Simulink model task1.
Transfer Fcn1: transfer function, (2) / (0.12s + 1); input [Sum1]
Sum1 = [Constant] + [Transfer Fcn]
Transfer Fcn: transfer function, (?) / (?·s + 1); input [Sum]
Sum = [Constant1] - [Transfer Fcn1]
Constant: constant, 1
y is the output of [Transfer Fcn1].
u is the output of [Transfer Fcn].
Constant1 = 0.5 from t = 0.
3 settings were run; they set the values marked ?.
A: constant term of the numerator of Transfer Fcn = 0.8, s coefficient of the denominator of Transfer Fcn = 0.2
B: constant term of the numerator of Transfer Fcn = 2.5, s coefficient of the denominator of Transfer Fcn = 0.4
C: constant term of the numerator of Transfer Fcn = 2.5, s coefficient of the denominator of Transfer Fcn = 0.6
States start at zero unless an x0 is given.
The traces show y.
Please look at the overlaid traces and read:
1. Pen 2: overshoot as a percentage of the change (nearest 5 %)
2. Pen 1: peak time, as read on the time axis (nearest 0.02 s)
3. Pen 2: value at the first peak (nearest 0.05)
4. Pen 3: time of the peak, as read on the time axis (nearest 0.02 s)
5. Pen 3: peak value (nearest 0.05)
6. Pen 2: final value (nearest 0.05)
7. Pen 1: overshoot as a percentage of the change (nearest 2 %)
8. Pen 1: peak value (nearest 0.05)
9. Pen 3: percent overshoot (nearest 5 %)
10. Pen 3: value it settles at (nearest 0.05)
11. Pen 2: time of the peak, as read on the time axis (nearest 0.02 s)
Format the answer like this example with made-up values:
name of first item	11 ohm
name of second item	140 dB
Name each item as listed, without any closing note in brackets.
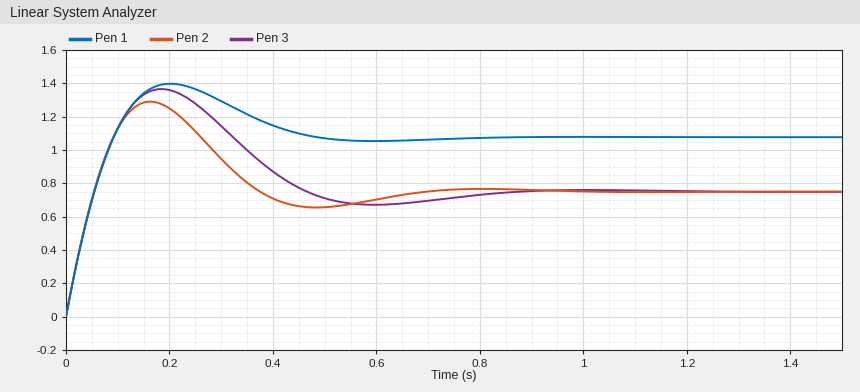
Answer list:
Pen 2: overshoot as a percentage of the change	70 %
Pen 1: peak time, as read on the time axis	0.20 s
Pen 2: value at the first peak	1.30
Pen 3: time of the peak, as read on the time axis	0.18 s
Pen 3: peak value	1.35
Pen 2: final value	0.75
Pen 1: overshoot as a percentage of the change	30 %
Pen 1: peak value	1.40
Pen 3: percent overshoot	80 %
Pen 3: value it settles at	0.75
Pen 2: time of the peak, as read on the time axis	0.16 s
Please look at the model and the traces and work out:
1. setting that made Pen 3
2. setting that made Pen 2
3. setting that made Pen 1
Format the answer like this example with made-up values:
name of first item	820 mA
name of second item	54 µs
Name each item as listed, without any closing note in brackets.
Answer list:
setting that made Pen 3	C
setting that made Pen 2	B
setting that made Pen 1	A
